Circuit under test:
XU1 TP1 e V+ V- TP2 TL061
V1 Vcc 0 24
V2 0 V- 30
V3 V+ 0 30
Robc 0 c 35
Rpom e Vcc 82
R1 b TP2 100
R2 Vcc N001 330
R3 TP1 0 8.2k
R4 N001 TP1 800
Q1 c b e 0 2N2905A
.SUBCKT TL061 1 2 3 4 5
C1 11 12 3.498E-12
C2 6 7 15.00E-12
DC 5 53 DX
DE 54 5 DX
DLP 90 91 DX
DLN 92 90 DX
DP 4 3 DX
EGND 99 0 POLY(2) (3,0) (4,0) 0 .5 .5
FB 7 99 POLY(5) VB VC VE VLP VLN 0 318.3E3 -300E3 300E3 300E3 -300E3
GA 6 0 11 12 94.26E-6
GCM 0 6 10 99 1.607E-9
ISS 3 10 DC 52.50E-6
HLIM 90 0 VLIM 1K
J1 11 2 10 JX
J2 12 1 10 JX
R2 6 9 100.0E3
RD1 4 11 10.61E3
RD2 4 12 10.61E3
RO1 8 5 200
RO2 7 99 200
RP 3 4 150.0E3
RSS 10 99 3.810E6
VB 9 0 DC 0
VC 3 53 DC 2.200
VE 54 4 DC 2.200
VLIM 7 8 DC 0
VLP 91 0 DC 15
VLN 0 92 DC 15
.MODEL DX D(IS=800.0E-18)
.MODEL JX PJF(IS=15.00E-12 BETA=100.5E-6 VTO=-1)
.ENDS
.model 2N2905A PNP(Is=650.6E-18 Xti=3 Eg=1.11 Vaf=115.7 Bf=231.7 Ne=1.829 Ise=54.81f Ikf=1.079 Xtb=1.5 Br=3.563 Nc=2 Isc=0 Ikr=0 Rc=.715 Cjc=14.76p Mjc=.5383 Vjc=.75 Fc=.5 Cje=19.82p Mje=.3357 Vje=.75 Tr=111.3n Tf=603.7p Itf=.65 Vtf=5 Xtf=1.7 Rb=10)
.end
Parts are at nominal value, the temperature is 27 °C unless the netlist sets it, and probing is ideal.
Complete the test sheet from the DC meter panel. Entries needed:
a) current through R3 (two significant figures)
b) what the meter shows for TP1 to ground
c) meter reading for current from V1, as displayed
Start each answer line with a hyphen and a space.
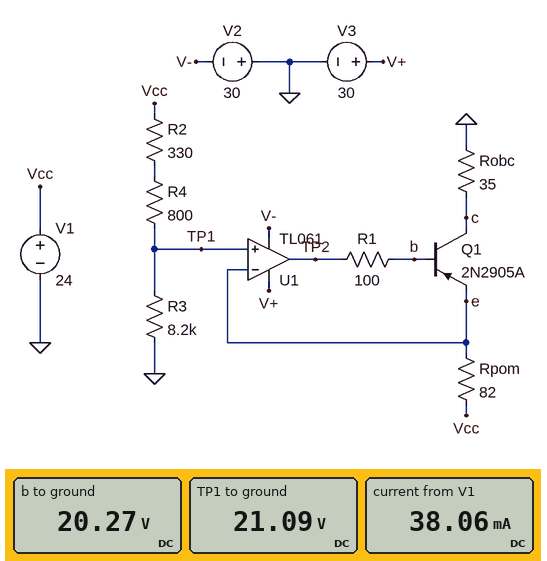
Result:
- 2.6 mA
- 21.09 V
- 38.06 mA
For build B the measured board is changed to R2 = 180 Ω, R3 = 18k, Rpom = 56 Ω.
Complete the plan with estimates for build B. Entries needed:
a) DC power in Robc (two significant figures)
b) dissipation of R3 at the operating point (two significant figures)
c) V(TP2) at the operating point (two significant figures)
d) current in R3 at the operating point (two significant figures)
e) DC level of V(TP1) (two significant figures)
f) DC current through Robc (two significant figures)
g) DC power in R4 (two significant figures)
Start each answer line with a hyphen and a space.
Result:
- 17 mW
- 29 mW
- 22 V
- 1.3 mA
- 23 V
- 22 mA
- 1.3 mW
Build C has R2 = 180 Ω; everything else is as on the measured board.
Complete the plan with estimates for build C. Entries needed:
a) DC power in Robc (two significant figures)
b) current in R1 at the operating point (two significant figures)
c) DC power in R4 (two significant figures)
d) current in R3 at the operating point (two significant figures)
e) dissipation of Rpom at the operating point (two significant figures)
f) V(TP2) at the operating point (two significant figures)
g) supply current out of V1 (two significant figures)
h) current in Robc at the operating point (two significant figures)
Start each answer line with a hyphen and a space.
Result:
- 34 mW
- 120 µA
- 5.5 mW
- 2.6 mA
- 80 mW
- 21 V
- 34 mA
- 31 mA
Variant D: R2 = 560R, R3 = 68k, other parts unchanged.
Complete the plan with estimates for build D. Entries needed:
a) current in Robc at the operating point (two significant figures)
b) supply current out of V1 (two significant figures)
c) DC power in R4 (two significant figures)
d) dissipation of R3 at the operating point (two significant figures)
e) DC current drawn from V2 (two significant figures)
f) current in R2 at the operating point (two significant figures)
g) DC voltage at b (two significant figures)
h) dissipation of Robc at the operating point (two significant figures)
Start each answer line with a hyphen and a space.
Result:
- 5.8 mA
- 6.1 mA
- 96 µW
- 8.1 mW
- 450 µA
- 350 µA
- 23 V
- 1.2 mW
